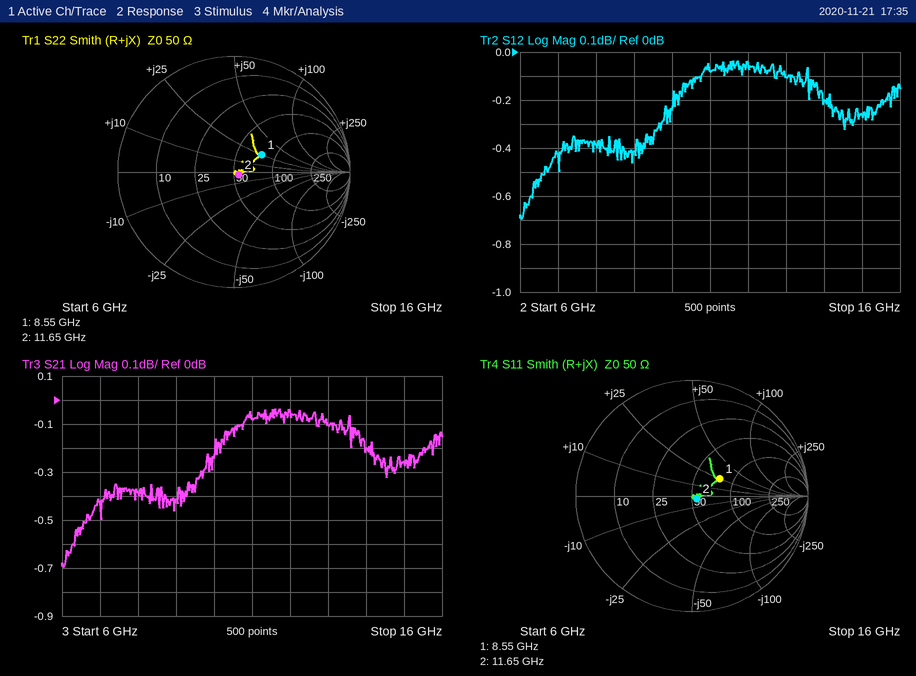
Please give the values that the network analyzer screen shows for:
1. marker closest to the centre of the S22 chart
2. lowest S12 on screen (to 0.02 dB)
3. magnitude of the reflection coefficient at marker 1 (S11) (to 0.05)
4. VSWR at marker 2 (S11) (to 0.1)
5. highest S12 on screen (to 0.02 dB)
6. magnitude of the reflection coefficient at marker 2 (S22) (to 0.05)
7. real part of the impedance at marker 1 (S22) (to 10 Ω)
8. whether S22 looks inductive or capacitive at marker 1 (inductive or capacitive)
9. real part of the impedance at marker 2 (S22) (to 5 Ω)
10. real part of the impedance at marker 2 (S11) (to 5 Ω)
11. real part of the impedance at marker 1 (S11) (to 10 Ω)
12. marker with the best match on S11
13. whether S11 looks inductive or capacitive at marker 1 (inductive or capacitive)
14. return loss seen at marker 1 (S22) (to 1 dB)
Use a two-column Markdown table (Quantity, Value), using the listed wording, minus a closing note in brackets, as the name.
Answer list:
| Quantity | Value |
|---|---|
| marker closest to the centre of the S22 chart | marker 2 |
| lowest S12 on screen | -0.70 dB |
| magnitude of the reflection coefficient at marker 1 (S11) | 0.30 |
| VSWR at marker 2 (S11) | 1.1 |
| highest S12 on screen | -0.04 dB |
| magnitude of the reflection coefficient at marker 2 (S22) | 0.05 |
| real part of the impedance at marker 1 (S22) | 80 Ω |
| whether S22 looks inductive or capacitive at marker 1 | inductive |
| real part of the impedance at marker 2 (S22) | 55 Ω |
| real part of the impedance at marker 2 (S11) | 55 Ω |
| real part of the impedance at marker 1 (S11) | 80 Ω |
| marker with the best match on S11 | marker 2 |
| whether S11 looks inductive or capacitive at marker 1 | inductive |
| return loss seen at marker 1 (S22) | 11 dB |
